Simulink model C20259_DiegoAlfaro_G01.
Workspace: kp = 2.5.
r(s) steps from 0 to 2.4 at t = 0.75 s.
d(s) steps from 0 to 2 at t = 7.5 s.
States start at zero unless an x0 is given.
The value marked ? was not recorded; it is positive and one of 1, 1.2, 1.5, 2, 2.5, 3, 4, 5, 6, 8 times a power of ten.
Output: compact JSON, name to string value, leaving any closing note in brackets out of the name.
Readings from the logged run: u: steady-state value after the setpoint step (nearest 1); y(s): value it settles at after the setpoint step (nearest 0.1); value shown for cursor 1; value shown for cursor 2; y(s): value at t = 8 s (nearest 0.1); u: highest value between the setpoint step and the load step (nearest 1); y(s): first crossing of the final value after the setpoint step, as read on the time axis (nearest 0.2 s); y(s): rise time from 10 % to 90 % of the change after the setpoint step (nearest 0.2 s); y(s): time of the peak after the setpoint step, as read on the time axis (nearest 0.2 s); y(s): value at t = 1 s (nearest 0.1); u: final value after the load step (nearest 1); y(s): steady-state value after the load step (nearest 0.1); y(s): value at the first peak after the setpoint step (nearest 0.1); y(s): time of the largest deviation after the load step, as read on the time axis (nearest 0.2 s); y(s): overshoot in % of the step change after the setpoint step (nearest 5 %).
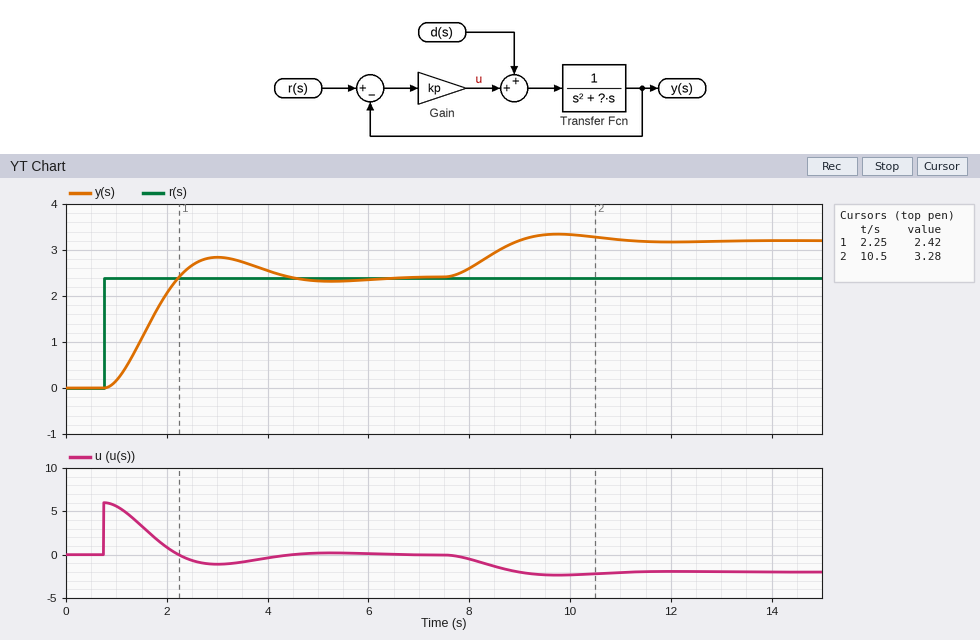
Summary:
{"u: steady-state value after the setpoint step": "0", "y(s): value it settles at after the setpoint step": "2.4", "value shown for cursor 1": "2.42", "value shown for cursor 2": "3.28", "y(s): value at t = 8 s": "2.6", "u: highest value between the setpoint step and the load step": "6", "y(s): first crossing of the final value after the setpoint step, as read on the time axis": "2.2 s", "y(s): rise time from 10 % to 90 % of the change after the setpoint step": "1.0 s", "y(s): time of the peak after the setpoint step, as read on the time axis": "3.0 s", "y(s): value at t = 1 s": "0.2", "u: final value after the load step": "-2", "y(s): steady-state value after the load step": "3.2", "y(s): value at the first peak after the setpoint step": "2.8", "y(s): time of the largest deviation after the load step, as read on the time axis": "9.8 s", "y(s): overshoot in % of the step change after the setpoint step": "20 %"}
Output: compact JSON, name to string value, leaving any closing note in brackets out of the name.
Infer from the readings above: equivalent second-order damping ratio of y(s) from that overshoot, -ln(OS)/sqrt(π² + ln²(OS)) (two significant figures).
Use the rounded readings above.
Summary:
{"equivalent second-order damping ratio of y(s) from that overshoot, -ln(OS)/sqrt(π² + ln²(OS))": "0.46"}
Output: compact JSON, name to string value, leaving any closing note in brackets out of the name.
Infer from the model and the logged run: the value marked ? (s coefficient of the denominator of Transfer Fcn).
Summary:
{"the value marked ?": "1.5"}
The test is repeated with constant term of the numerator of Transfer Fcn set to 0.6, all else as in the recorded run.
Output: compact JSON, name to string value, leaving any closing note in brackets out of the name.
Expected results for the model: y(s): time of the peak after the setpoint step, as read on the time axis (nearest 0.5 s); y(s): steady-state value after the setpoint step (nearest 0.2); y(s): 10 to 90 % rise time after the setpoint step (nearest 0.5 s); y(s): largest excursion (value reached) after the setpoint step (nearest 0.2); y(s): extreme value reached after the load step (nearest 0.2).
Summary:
{"y(s): time of the peak after the setpoint step, as read on the time axis": "4.0 s", "y(s): steady-state value after the setpoint step": "2.4", "y(s): 10 to 90 % rise time after the setpoint step": "1.5 s", "y(s): largest excursion (value reached) after the setpoint step": "2.6", "y(s): extreme value reached after the load step": "3.2"}
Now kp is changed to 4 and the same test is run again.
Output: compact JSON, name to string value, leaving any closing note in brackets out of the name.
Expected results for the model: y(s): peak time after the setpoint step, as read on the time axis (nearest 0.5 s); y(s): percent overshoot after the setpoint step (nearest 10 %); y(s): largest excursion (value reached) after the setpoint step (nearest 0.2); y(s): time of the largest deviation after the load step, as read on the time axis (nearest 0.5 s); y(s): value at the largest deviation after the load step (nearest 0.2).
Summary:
{"y(s): peak time after the setpoint step, as read on the time axis": "2.5 s", "y(s): percent overshoot after the setpoint step": "30 %", "y(s): largest excursion (value reached) after the setpoint step": "3.0", "y(s): time of the largest deviation after the load step, as read on the time axis": "9.0 s", "y(s): value at the largest deviation after the load step": "3.0"}
